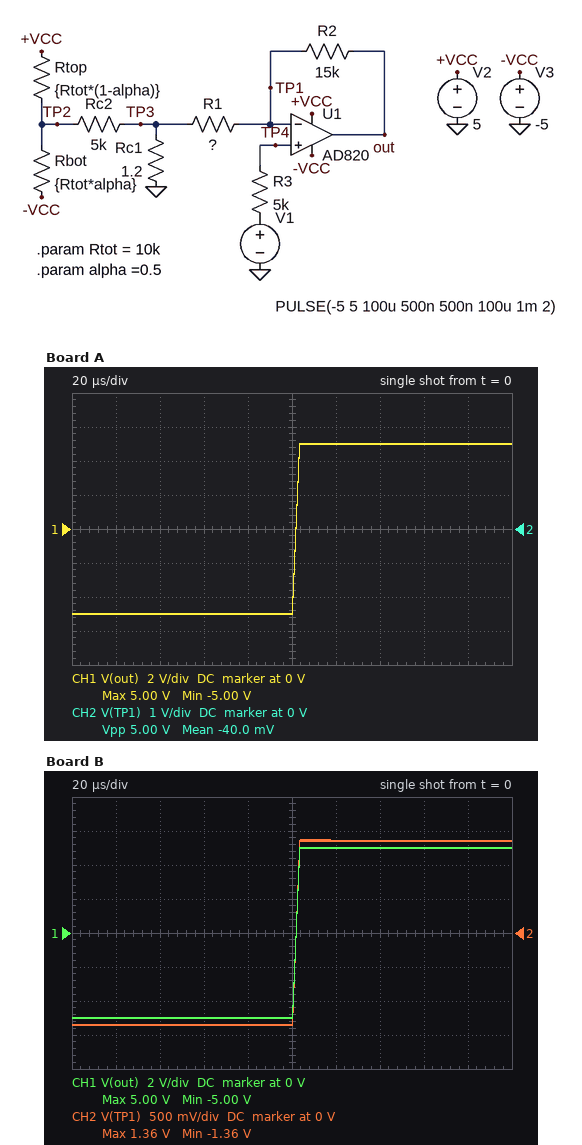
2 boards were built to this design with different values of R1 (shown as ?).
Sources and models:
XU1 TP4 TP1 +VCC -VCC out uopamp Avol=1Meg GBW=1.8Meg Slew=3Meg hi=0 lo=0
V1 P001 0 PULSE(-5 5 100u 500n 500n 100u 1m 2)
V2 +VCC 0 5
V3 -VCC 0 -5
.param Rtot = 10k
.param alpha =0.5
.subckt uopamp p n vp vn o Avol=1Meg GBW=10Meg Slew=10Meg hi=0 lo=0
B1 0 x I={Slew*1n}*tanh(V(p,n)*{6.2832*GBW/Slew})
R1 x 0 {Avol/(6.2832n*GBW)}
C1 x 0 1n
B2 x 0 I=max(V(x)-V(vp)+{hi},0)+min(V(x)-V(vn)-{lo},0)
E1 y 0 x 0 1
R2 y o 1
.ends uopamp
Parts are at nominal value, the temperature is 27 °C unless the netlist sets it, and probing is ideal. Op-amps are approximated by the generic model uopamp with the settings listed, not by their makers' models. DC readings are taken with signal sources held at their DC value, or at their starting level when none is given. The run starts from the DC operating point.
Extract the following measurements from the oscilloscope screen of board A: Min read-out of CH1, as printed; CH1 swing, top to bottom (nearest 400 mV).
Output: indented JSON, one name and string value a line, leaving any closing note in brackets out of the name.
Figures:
{
  "Min read-out of CH1, as printed": "-5.00 V",
  "CH1 swing, top to bottom": "10.0 V"
}
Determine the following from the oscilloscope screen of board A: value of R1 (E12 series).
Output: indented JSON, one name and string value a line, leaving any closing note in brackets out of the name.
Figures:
{
  "value of R1": "15 kΩ"
}
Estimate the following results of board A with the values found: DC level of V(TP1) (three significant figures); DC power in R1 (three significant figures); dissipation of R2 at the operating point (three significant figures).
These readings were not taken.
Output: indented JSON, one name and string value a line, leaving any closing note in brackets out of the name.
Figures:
{
  "DC level of V(TP1)": "-2.50 V",
  "DC power in R1": "417 µW",
  "dissipation of R2 at the operating point": "417 µW"
}
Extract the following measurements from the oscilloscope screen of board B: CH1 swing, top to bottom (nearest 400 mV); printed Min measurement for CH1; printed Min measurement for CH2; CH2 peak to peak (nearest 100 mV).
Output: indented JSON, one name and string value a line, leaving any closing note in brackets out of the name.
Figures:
{
  "CH1 swing, top to bottom": "10.0 V",
  "printed Min measurement for CH1": "-5.00 V",
  "printed Min measurement for CH2": "-1.36 V",
  "CH2 peak to peak": "2.7 V"
}
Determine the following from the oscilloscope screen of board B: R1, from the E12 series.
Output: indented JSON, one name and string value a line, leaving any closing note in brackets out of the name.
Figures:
{
  "R1, from the E12 series": "5.6 kΩ"
}
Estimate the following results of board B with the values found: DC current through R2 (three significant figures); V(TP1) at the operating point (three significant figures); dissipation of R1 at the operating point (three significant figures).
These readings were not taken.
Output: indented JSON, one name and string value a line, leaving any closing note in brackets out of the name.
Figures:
{
  "DC current through R2": "243 µA",
  "V(TP1) at the operating point": "-1.36 V",
  "dissipation of R1 at the operating point": "330 µW"
}
